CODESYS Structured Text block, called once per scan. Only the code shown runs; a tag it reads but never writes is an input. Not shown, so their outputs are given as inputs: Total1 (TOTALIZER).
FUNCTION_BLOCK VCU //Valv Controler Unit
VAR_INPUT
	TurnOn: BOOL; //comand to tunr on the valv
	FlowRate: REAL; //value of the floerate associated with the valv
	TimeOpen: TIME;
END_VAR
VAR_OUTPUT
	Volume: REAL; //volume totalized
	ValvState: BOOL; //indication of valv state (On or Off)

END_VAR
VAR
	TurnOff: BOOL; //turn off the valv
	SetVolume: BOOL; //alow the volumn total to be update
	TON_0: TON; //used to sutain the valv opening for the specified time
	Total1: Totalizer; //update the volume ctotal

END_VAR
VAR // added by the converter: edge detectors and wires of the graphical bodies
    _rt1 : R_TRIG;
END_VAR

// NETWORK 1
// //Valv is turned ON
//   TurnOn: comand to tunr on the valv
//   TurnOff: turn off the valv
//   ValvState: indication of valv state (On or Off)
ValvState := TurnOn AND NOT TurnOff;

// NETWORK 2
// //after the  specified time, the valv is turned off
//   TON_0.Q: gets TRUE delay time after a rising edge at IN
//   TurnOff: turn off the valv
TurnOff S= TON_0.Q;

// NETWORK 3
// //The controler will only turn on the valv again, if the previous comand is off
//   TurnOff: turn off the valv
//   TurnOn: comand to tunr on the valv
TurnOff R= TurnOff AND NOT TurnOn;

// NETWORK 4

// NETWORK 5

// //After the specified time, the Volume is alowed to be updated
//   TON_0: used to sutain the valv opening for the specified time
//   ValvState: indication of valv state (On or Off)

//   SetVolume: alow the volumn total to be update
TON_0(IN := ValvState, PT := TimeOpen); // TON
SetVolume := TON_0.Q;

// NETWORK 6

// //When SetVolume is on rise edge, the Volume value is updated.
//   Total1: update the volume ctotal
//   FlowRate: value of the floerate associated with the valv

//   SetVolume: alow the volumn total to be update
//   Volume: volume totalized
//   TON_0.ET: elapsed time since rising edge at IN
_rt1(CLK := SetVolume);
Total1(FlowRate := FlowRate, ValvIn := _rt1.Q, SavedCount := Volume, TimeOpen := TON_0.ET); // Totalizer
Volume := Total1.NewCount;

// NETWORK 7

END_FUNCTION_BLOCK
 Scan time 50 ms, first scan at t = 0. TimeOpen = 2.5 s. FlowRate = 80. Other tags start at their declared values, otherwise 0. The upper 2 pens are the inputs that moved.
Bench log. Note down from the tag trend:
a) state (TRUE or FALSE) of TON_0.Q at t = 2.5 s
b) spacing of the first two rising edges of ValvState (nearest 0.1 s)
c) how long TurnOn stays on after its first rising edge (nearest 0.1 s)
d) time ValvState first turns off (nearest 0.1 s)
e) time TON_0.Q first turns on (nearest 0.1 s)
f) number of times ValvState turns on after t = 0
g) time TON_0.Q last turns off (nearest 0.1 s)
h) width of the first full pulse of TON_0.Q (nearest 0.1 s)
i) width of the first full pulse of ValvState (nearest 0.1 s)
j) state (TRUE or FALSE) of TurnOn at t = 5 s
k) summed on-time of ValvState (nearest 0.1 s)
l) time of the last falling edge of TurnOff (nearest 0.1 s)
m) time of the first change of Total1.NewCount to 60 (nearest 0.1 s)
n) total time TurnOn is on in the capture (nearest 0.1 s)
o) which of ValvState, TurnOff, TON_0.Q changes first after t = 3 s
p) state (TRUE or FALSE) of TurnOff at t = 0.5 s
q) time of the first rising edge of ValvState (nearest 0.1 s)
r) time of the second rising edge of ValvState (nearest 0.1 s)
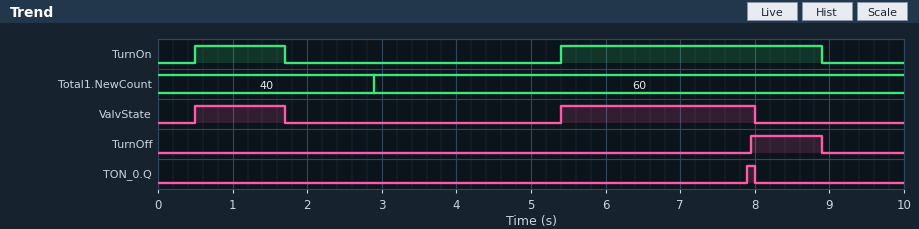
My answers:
FALSE
4.9 s
1.2 s
1.7 s
7.9 s
2
8.0 s
0.1 s
1.2 s
FALSE
3.8 s
8.9 s
2.9 s
4.7 s
ValvState
FALSE
0.5 s
5.4 s
